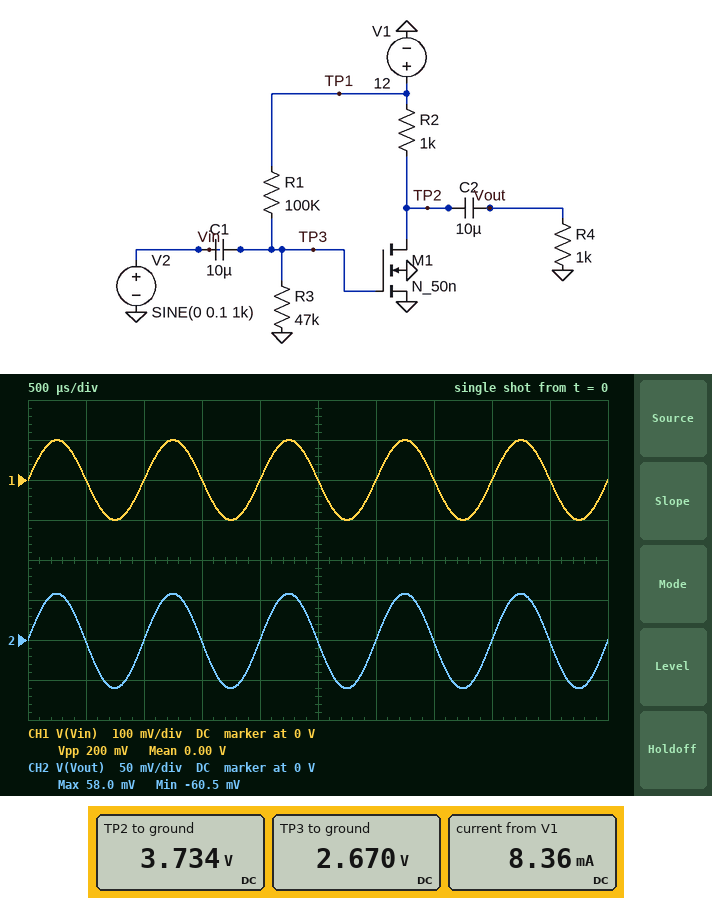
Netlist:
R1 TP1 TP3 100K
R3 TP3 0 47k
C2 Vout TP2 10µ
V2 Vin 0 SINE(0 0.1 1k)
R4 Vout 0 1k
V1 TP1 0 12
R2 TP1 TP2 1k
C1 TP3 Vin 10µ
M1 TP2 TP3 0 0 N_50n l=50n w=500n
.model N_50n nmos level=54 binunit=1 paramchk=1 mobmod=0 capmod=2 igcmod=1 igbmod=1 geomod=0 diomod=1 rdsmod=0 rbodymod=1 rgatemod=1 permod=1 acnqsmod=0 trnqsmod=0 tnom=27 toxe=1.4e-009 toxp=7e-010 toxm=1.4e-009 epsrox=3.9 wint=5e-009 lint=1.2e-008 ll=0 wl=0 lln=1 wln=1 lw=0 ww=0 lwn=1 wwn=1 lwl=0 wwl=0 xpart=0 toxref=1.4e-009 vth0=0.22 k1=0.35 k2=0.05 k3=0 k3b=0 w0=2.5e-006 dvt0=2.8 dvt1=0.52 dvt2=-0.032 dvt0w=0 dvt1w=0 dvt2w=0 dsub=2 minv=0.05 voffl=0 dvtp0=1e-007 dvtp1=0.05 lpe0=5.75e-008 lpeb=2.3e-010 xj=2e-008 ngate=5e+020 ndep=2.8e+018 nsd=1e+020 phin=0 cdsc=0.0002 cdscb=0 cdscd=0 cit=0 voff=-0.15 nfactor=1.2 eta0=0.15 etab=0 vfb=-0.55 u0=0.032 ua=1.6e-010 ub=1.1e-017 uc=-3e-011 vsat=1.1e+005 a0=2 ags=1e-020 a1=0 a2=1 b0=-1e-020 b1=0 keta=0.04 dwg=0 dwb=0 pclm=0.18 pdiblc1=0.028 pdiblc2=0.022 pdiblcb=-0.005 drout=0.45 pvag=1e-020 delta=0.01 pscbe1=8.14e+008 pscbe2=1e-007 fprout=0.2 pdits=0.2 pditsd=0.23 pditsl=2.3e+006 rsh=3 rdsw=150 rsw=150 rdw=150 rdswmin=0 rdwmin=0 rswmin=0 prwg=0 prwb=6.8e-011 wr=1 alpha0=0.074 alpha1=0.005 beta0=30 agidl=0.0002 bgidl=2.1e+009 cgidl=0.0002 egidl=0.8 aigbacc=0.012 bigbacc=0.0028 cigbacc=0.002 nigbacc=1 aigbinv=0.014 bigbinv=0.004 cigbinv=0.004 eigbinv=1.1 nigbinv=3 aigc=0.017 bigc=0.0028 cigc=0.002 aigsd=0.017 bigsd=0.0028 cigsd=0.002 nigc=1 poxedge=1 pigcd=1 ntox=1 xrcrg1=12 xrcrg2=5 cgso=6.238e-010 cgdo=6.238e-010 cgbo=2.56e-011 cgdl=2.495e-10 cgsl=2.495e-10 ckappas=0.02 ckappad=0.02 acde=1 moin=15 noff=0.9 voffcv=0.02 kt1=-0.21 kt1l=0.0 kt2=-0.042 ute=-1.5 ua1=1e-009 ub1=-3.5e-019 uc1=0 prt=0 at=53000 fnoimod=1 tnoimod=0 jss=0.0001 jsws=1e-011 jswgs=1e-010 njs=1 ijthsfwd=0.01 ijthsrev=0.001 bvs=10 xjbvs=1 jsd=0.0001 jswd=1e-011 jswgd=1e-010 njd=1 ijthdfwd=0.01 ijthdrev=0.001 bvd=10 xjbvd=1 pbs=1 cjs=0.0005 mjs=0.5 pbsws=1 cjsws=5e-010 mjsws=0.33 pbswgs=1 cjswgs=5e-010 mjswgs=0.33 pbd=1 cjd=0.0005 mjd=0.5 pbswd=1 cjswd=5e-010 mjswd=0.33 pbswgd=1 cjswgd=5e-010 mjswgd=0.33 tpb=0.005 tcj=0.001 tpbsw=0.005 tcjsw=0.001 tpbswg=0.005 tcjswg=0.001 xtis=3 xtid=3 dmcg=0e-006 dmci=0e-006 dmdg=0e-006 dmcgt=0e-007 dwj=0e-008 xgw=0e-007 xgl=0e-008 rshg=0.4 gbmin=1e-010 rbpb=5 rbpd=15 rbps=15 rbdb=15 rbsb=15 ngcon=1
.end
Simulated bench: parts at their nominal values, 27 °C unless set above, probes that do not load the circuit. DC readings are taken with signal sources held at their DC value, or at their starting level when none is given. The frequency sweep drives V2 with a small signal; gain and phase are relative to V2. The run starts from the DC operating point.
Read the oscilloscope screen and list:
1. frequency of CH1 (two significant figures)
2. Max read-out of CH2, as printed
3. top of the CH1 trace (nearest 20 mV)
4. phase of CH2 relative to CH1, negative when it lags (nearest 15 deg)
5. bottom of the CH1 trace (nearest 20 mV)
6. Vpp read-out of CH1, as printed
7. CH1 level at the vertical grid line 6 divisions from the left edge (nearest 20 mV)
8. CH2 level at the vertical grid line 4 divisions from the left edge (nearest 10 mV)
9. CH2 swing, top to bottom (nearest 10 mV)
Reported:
1.0 kHz
58.0 mV
100 mV
0 deg
-100 mV
200 mV
0 V
0 V
120 mV
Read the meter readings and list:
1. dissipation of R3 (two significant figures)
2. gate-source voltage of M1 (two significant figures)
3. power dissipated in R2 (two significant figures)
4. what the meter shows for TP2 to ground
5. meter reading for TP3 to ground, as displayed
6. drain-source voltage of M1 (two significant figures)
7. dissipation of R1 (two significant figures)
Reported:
150 µW
2.7 V
68 mW
3.734 V
2.670 V
3.7 V
870 µW
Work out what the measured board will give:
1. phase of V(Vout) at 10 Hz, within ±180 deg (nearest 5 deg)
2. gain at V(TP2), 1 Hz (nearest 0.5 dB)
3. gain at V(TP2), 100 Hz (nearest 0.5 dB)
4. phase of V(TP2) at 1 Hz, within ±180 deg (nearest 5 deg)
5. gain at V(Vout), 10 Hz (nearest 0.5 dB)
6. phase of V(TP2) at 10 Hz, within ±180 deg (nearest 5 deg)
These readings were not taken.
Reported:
80 deg
-16.5 dB
-4.5 dB
75 deg
-10.5 dB
20 deg
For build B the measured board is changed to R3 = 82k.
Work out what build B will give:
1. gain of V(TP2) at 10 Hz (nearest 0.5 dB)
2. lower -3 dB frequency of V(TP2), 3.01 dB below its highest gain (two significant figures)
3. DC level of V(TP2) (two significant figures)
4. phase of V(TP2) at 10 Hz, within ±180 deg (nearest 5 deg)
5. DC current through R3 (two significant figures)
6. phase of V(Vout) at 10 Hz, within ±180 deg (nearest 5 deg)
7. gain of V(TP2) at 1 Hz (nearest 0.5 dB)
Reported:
-5.5 dB
5.5 Hz
3.8 V
30 deg
34 µA
85 deg
-19.5 dB
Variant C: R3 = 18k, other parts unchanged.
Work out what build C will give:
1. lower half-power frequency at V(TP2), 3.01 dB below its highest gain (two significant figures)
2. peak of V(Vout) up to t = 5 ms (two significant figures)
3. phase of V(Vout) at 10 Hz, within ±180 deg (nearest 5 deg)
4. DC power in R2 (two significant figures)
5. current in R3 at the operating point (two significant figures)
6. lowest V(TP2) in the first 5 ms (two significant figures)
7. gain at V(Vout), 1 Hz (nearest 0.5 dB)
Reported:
1.0 Hz
55 mV
65 deg
77 mW
100 µA
3.2 V
-32.5 dB
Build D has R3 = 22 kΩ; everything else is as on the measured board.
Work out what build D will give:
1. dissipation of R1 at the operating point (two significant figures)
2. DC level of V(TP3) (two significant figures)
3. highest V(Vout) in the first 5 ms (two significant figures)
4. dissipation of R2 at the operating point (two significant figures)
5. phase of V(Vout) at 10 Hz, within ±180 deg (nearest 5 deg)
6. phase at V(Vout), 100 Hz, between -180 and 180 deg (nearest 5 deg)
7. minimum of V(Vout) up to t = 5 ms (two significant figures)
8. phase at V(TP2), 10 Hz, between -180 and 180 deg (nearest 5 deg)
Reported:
970 µW
2.1 V
57 mV
74 mW
65 deg
10 deg
-58 mV
5 deg
